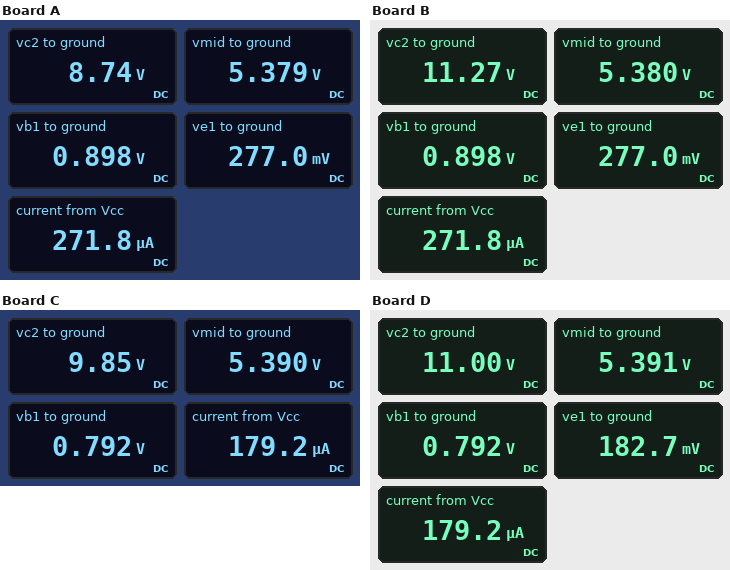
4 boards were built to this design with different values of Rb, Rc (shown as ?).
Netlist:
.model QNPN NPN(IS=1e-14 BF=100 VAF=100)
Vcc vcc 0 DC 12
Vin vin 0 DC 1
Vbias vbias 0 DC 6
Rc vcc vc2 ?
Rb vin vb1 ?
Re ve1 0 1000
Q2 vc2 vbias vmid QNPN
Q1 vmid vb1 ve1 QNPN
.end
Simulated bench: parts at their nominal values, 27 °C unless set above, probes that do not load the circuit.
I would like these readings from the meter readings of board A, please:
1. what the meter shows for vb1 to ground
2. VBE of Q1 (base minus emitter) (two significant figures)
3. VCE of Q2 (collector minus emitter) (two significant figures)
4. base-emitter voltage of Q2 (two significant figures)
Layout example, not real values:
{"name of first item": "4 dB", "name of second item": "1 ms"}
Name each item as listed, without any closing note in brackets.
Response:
{"what the meter shows for vb1 to ground": "0.898 V", "VBE of Q1 (base minus emitter)": "620 mV", "VCE of Q2 (collector minus emitter)": "3.4 V", "base-emitter voltage of Q2": "620 mV"}
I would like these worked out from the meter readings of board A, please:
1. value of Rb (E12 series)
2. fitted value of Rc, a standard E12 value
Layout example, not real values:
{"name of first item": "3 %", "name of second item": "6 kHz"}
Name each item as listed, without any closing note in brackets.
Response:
{"value of Rb": "39 kΩ", "fitted value of Rc, a standard E12 value": "12 kΩ"}
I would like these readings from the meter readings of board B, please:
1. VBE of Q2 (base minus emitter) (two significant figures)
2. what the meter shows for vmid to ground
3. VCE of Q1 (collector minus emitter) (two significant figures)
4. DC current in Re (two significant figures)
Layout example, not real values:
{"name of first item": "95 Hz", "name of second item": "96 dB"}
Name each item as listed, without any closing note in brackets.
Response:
{"VBE of Q2 (base minus emitter)": "620 mV", "what the meter shows for vmid to ground": "5.380 V", "VCE of Q1 (collector minus emitter)": "5.1 V", "DC current in Re": "280 µA"}
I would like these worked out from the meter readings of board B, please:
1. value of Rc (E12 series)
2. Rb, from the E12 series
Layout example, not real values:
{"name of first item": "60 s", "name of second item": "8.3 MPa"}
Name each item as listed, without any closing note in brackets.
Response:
{"value of Rc": "2.7 kΩ", "Rb, from the E12 series": "39 kΩ"}
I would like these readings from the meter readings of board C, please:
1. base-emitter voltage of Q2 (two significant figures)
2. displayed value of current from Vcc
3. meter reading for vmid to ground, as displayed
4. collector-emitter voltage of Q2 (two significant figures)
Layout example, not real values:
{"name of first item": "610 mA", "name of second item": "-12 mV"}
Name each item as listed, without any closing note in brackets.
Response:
{"base-emitter voltage of Q2": "610 mV", "displayed value of current from Vcc": "179.2 µA", "meter reading for vmid to ground, as displayed": "5.390 V", "collector-emitter voltage of Q2": "4.5 V"}
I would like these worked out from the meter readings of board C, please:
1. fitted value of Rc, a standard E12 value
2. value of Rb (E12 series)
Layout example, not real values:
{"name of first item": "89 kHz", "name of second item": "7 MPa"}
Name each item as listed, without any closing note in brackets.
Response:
{"fitted value of Rc, a standard E12 value": "12 kΩ", "value of Rb": "120 kΩ"}
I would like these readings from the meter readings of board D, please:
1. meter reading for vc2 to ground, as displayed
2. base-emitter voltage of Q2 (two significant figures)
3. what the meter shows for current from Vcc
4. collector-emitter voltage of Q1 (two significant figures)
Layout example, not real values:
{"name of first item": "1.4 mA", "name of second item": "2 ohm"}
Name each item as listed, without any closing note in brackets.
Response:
{"meter reading for vc2 to ground, as displayed": "11.00 V", "base-emitter voltage of Q2": "610 mV", "what the meter shows for current from Vcc": "179.2 µA", "collector-emitter voltage of Q1": "5.2 V"}
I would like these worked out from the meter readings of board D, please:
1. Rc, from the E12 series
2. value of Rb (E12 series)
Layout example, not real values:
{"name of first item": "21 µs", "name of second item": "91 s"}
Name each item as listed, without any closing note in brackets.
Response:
{"Rc, from the E12 series": "5.6 kΩ", "value of Rb": "120 kΩ"}
